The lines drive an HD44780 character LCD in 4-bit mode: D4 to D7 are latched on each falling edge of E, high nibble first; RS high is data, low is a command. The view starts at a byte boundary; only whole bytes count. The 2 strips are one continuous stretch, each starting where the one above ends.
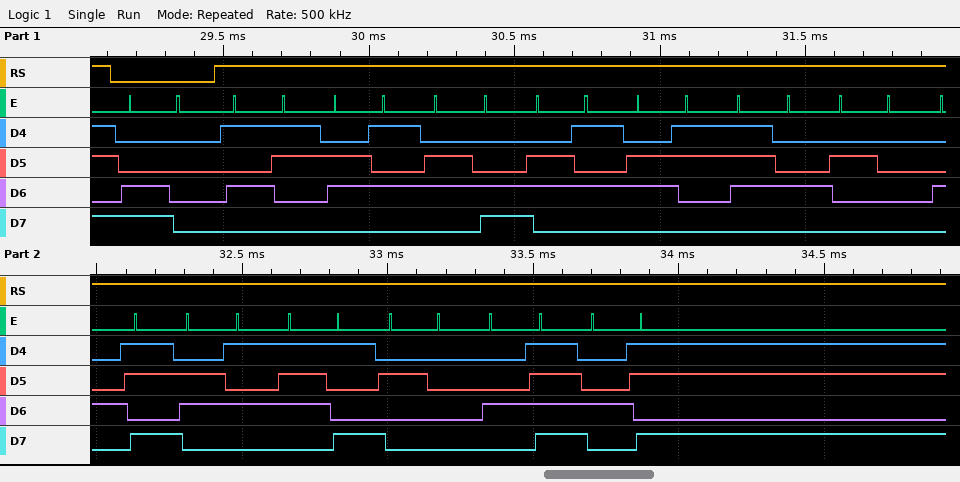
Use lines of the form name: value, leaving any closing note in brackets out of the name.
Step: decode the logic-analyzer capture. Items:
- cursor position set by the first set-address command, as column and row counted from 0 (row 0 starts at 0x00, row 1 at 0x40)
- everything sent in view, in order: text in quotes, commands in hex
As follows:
cursor position set by the first set-address command, as column and row counted from 0: column 0, row 1
everything sent in view, in order: text in quotes, commands in hex: 0xC0 "Select Key OK"
